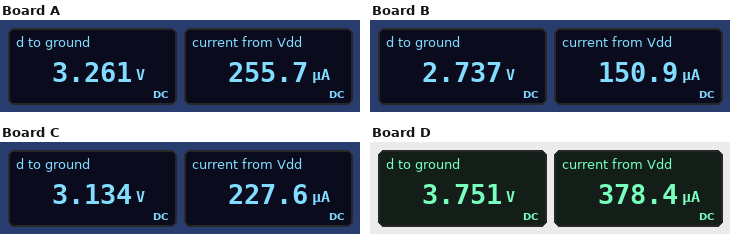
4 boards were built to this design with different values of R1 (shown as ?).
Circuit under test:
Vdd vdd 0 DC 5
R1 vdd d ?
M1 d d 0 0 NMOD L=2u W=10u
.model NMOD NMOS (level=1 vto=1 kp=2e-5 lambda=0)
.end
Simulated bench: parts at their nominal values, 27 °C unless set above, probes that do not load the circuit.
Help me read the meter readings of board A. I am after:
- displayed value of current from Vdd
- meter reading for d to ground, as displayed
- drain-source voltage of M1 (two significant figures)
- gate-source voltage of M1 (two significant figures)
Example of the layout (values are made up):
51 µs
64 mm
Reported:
255.7 µA
3.261 V
3.3 V
3.3 V
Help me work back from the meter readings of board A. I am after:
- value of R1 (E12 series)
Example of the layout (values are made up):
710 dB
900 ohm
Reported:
6.8 kΩ
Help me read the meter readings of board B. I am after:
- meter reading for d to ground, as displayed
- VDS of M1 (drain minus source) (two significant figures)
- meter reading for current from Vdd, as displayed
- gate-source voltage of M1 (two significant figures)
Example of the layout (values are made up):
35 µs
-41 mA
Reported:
2.737 V
2.7 V
150.9 µA
2.7 V
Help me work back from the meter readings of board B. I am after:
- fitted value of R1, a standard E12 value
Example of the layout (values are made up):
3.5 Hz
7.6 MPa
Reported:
15 kΩ
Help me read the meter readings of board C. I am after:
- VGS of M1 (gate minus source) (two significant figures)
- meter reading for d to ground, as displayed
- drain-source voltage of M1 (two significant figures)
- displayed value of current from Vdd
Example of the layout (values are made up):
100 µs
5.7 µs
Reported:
3.1 V
3.134 V
3.1 V
227.6 µA
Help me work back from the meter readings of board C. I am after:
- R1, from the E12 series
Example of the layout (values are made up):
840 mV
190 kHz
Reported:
8.2 kΩ
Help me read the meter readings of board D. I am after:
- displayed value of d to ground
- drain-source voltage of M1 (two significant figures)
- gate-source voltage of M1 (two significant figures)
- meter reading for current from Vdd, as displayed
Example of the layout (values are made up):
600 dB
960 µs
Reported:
3.751 V
3.8 V
3.8 V
378.4 µA
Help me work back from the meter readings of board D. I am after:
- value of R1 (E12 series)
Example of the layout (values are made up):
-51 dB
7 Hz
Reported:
3.3 kΩ
